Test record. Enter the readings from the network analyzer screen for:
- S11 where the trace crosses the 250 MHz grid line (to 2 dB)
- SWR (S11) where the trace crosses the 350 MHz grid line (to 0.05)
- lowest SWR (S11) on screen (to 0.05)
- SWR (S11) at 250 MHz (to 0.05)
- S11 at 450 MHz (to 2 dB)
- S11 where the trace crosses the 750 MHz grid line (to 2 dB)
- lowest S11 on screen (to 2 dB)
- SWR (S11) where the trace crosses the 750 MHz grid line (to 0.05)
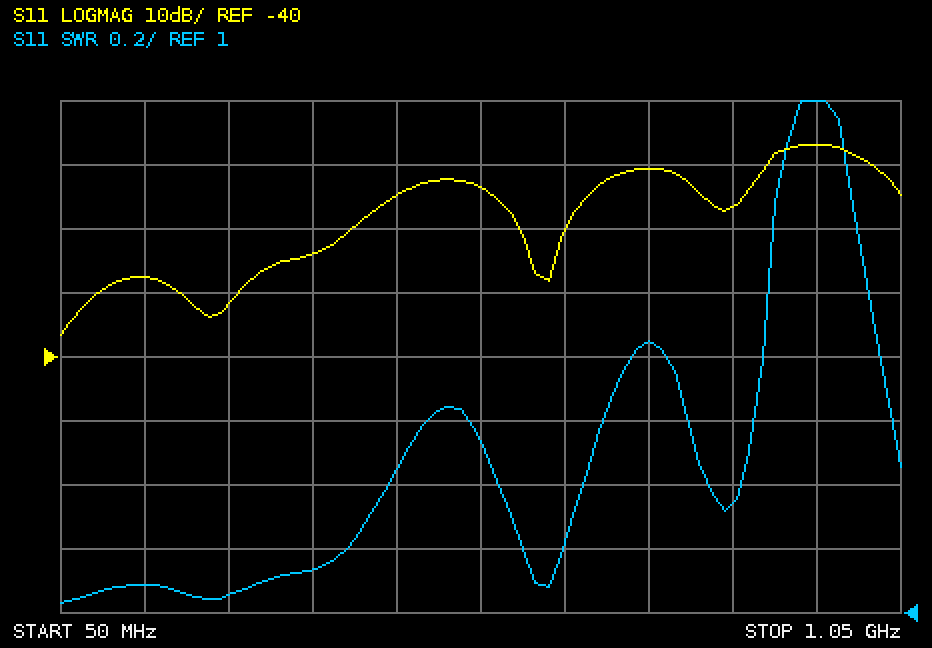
-32 dB
1.15
1.05
1.05
-14 dB
-10 dB
-36 dB
1.85
